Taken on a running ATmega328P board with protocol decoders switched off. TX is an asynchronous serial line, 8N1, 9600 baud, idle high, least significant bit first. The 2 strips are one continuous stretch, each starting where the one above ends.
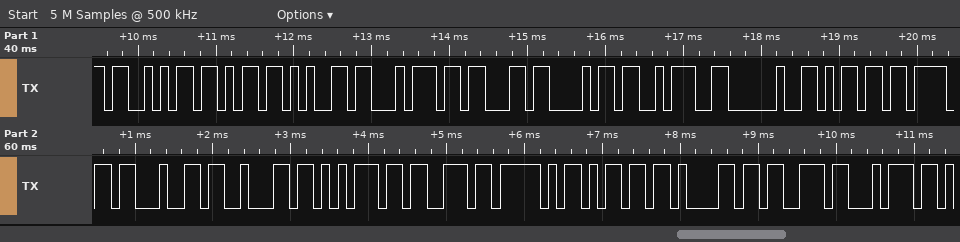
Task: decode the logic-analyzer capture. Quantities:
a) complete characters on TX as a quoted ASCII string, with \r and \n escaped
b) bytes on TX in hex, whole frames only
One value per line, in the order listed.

"Sketch: modbus_mast"
0x53 0x6B 0x65 0x74 0x63 0x68 0x3A 0x20 0x6D 0x6F 0x64 0x62 0x75 0x73 0x5F 0x6D 0x61 0x73 0x74
